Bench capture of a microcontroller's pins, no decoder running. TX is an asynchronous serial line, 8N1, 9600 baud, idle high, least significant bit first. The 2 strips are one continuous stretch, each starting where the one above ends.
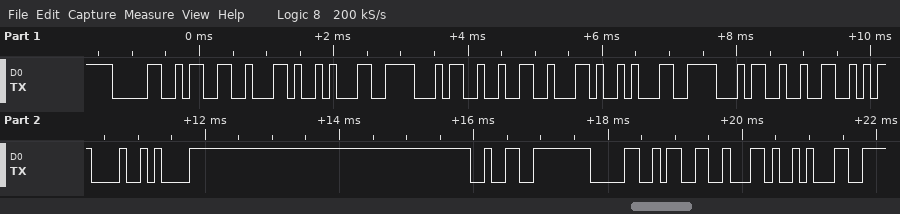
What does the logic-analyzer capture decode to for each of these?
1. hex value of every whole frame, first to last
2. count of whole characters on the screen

30 33 2C 31 34 32 2C 31 34 32 0D 0A 32 30 33 2C 31
17
